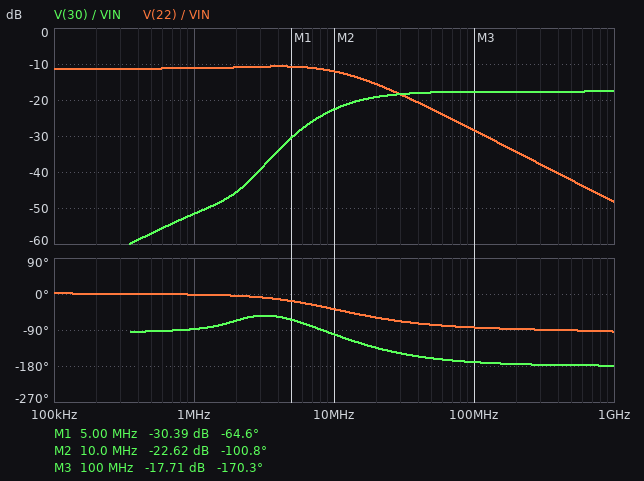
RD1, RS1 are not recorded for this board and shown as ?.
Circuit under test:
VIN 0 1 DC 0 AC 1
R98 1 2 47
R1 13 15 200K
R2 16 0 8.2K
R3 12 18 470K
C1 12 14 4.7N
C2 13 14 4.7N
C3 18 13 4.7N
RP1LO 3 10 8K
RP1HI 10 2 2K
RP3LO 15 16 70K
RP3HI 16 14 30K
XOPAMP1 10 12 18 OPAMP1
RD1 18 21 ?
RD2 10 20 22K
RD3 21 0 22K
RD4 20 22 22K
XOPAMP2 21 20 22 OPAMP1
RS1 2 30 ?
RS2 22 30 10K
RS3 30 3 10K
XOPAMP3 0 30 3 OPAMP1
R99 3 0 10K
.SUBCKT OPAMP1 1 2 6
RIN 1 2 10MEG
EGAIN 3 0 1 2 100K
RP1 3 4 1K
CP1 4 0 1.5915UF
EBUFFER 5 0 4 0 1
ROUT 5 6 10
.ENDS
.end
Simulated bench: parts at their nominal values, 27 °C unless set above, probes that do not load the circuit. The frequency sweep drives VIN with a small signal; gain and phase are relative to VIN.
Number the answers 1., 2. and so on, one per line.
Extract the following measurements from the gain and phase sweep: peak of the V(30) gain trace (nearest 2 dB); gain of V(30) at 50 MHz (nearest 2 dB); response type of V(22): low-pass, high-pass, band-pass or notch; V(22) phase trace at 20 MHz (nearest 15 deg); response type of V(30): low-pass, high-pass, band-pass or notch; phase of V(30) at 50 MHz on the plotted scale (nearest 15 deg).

1. -18 dB
2. -18 dB
3. low-pass
4. -60 deg
5. high-pass
6. -165 deg
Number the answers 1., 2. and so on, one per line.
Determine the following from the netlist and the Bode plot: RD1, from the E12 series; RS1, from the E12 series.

1. 47 kΩ
2. 33 kΩ
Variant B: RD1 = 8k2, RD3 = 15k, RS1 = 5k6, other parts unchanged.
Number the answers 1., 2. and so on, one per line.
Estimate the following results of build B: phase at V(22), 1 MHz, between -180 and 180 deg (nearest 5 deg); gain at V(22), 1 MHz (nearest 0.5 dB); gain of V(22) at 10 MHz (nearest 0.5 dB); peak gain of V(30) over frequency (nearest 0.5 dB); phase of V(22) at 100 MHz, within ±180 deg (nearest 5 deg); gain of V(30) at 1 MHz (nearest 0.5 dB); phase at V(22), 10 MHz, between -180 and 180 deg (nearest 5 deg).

1. 160 deg
2. -17.0 dB
3. -12.5 dB
4. -6.5 dB
5. -80 deg
6. -15.0 dB
7. 5 deg
